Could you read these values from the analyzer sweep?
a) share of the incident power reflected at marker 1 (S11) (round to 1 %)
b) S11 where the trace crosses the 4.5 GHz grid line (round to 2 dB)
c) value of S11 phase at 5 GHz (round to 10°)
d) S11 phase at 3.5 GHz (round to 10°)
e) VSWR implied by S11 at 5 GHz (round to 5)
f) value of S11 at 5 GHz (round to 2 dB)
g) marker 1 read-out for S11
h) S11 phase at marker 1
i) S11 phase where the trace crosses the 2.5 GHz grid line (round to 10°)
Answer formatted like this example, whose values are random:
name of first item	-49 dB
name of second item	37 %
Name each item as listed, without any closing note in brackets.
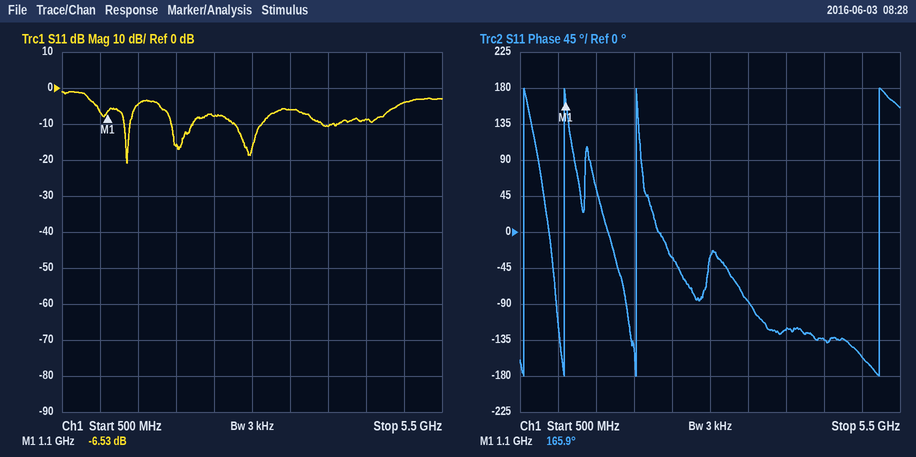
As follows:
share of the incident power reflected at marker 1 (S11)	22 %
S11 where the trace crosses the 4.5 GHz grid line	-8 dB
value of S11 phase at 5 GHz	-160°
S11 phase at 3.5 GHz	-90°
VSWR implied by S11 at 5 GHz	5
value of S11 at 5 GHz	-4 dB
marker 1 read-out for S11	-6.53 dB
S11 phase at marker 1	165.9°
S11 phase where the trace crosses the 2.5 GHz grid line	-30°
